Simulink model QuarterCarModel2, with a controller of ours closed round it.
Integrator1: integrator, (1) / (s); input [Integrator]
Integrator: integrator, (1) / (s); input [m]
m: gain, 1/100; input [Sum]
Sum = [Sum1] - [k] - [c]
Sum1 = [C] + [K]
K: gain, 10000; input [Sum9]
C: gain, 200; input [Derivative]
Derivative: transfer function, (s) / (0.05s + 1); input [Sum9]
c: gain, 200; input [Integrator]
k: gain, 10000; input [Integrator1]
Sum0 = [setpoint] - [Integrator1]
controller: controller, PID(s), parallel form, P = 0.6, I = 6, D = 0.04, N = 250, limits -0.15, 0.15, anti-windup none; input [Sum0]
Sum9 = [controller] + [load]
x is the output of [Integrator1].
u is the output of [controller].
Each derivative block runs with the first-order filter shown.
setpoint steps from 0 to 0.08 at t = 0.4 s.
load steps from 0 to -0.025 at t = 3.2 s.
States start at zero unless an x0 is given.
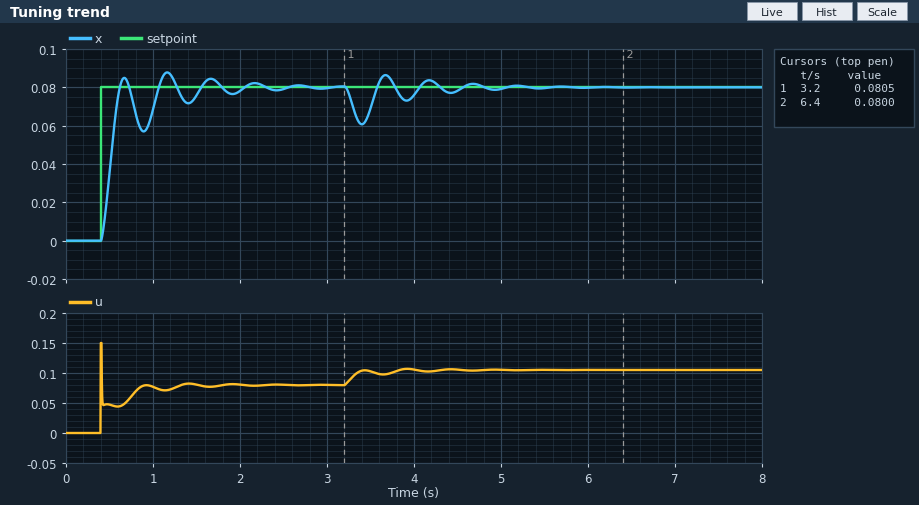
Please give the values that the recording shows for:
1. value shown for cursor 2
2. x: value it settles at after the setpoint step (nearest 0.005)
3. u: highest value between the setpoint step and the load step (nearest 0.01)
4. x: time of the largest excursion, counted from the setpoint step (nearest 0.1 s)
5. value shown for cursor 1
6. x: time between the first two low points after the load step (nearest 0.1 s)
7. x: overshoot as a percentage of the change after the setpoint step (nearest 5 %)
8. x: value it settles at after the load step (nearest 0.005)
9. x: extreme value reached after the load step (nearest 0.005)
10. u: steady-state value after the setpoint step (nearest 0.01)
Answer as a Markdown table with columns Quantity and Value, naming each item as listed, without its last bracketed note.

| Quantity | Value |
|---|---|
| value shown for cursor 2 | 0.0800 |
| x: value it settles at after the setpoint step | 0.080 |
| u: highest value between the setpoint step and the load step | 0.15 |
| x: time of the largest excursion, counted from the setpoint step | 0.8 s |
| value shown for cursor 1 | 0.0805 |
| x: time between the first two low points after the load step | 0.5 s |
| x: overshoot as a percentage of the change after the setpoint step | 10 % |
| x: value it settles at after the load step | 0.080 |
| x: extreme value reached after the load step | 0.060 |
| u: steady-state value after the setpoint step | 0.08 |
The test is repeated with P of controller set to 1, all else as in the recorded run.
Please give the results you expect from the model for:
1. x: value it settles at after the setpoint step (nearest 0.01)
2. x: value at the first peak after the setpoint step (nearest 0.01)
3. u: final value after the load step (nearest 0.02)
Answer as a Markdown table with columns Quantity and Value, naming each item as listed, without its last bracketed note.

| Quantity | Value |
|---|---|
| x: value it settles at after the setpoint step | 0.08 |
| x: value at the first peak after the setpoint step | 0.09 |
| u: final value after the load step | 0.10 |
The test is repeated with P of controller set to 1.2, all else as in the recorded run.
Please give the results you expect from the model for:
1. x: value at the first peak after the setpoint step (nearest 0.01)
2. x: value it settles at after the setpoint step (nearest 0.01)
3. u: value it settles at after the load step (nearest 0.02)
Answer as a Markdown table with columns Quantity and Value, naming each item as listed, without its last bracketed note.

| Quantity | Value |
|---|---|
| x: value at the first peak after the setpoint step | 0.09 |
| x: value it settles at after the setpoint step | 0.08 |
| u: value it settles at after the load step | 0.10 |
